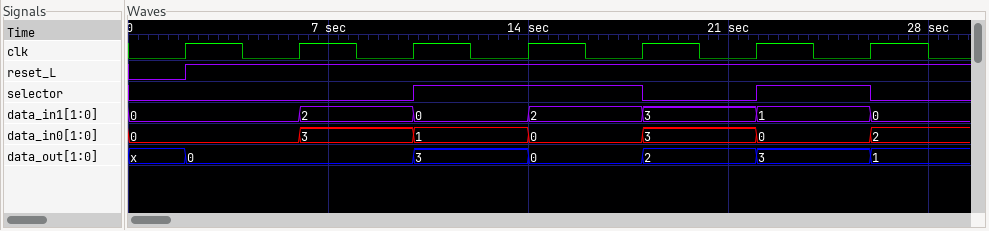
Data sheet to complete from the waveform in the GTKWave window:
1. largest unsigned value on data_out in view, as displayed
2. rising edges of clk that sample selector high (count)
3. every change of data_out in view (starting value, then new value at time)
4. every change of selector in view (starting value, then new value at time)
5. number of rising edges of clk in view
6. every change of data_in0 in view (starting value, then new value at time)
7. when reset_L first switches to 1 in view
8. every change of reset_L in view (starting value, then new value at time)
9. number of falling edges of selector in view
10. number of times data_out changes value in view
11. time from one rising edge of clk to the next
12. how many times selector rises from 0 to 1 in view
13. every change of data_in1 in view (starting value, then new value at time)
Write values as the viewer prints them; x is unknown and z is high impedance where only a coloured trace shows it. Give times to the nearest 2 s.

3
3
x, 0 at 2 s, 3 at 10 s, 0 at 14 s, 2 at 18 s, 3 at 22 s, 1 at 26 s
0, 1 at 10 s, 0 at 18 s, 1 at 22 s, 0 at 26 s
7
0, 3 at 6 s, 1 at 10 s, 0 at 14 s, 3 at 18 s, 0 at 22 s, 2 at 26 s
2 s
0, 1 at 2 s
2
6
4 s
2
0, 2 at 6 s, 0 at 10 s, 2 at 14 s, 3 at 18 s, 1 at 22 s, 0 at 26 s
